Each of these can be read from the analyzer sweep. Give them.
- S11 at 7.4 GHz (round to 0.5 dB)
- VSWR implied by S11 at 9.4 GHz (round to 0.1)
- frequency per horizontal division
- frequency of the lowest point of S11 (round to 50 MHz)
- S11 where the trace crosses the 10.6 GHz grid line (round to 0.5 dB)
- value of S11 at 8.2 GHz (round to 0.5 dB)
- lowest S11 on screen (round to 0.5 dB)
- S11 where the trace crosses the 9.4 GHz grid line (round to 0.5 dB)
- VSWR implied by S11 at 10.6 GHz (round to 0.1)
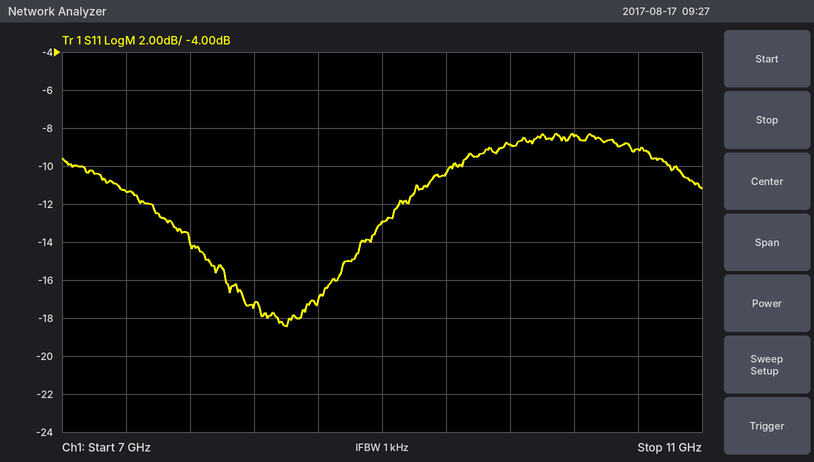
-11.5 dB
1.9
400 MHz
8.40 GHz
-9.0 dB
-17.5 dB
-18.5 dB
-10.5 dB
2.1
